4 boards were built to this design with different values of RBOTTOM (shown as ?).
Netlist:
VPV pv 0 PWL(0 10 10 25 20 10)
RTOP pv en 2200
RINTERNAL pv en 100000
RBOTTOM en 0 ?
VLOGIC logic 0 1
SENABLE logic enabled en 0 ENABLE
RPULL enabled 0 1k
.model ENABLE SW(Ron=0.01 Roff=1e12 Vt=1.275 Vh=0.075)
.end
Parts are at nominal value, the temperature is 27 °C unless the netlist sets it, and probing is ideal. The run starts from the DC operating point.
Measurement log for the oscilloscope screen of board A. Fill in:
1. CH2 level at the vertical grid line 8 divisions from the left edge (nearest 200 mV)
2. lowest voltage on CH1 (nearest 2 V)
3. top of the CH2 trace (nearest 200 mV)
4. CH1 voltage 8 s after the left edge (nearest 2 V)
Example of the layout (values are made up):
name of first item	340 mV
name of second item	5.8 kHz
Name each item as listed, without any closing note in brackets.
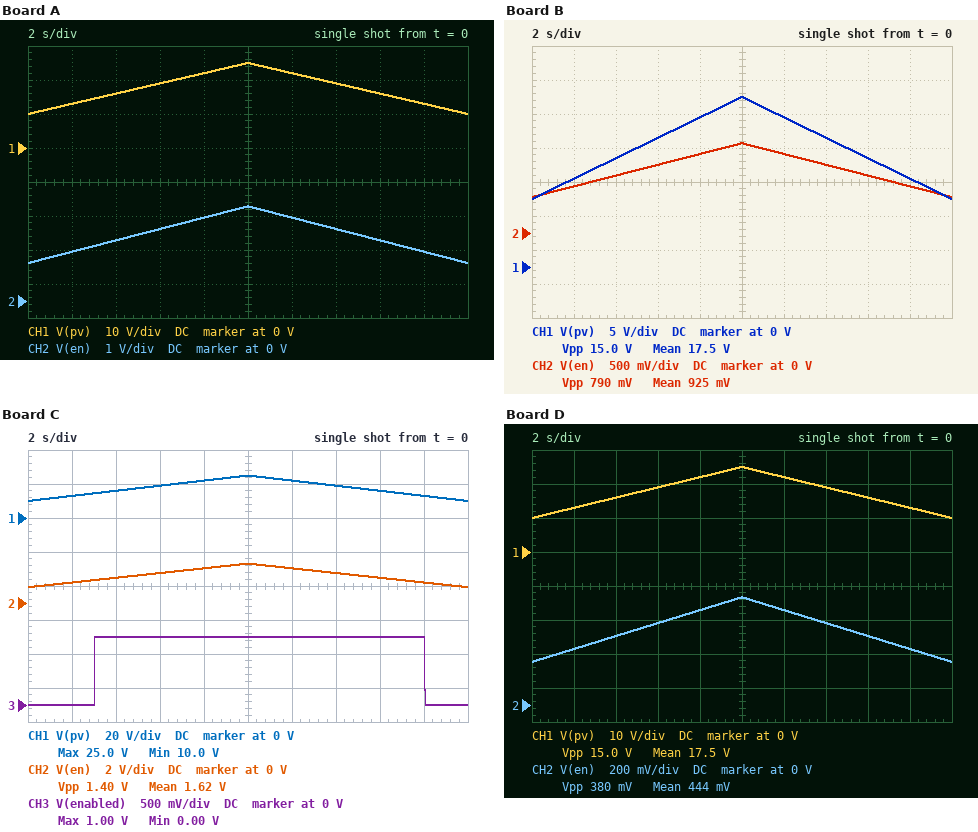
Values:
CH2 level at the vertical grid line 8 divisions from the left edge	1.8 V
lowest voltage on CH1	10 V
top of the CH2 trace	2.8 V
CH1 voltage 8 s after the left edge	22 V
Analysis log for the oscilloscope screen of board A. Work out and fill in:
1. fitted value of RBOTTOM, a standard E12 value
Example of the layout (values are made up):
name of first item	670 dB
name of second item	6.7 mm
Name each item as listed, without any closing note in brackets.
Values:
fitted value of RBOTTOM, a standard E12 value	270 Ω
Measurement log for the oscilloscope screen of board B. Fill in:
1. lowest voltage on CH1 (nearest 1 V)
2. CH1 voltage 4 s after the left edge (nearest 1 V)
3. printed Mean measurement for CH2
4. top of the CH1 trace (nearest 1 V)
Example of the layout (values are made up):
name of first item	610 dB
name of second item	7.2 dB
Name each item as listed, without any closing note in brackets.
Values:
lowest voltage on CH1	10 V
CH1 voltage 4 s after the left edge	16 V
printed Mean measurement for CH2	925 mV
top of the CH1 trace	25 V
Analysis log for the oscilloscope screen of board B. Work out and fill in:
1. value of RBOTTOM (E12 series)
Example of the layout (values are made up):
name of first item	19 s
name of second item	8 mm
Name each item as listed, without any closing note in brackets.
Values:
value of RBOTTOM	120 Ω
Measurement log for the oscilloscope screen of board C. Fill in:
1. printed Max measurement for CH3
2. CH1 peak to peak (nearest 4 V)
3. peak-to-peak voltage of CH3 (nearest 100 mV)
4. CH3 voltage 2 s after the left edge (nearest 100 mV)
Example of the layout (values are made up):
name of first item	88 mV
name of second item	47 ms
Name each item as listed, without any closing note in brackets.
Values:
printed Max measurement for CH3	1.00 V
CH1 peak to peak	16 V
peak-to-peak voltage of CH3	1.0 V
CH3 voltage 2 s after the left edge	0 V
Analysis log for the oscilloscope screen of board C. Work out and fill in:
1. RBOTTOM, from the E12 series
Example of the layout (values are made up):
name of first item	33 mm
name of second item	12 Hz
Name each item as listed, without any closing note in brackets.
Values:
RBOTTOM, from the E12 series	220 Ω
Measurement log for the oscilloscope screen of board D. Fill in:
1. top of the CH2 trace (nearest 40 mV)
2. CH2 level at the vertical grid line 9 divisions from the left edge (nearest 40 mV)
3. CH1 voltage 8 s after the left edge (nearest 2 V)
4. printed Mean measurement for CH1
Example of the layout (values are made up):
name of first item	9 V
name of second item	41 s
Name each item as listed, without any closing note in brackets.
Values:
top of the CH2 trace	640 mV
CH2 level at the vertical grid line 9 divisions from the left edge	320 mV
CH1 voltage 8 s after the left edge	22 V
printed Mean measurement for CH1	17.5 V
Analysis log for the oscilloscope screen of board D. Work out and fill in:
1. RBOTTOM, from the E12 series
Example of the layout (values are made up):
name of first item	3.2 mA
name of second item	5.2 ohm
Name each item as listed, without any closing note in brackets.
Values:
RBOTTOM, from the E12 series	56 Ω
